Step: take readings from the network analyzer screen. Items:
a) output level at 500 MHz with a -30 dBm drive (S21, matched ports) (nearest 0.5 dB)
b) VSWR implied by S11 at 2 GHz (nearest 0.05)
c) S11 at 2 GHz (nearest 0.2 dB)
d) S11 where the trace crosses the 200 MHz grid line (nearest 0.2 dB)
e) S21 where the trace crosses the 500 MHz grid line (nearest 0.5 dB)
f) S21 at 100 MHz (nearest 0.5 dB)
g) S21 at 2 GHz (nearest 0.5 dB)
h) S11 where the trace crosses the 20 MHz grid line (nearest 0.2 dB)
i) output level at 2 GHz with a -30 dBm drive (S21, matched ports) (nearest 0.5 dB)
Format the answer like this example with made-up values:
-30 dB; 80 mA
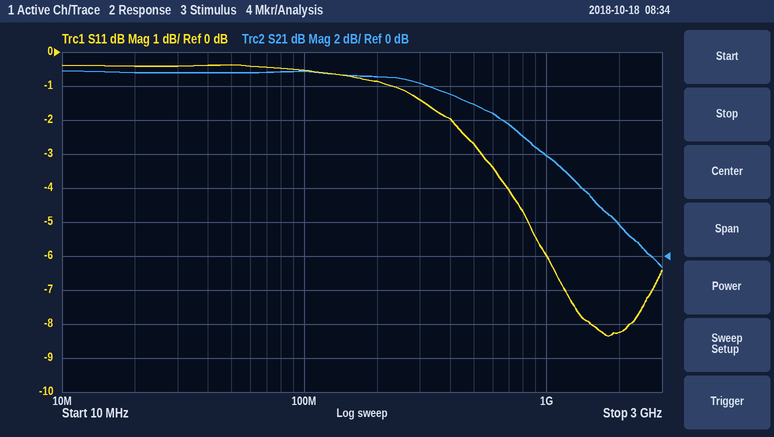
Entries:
-21.0 dBm; 2.25; -8.2 dB; -0.8 dB; 9.0 dB; 11.0 dB; 2.0 dB; -0.4 dB; -28.0 dBm
